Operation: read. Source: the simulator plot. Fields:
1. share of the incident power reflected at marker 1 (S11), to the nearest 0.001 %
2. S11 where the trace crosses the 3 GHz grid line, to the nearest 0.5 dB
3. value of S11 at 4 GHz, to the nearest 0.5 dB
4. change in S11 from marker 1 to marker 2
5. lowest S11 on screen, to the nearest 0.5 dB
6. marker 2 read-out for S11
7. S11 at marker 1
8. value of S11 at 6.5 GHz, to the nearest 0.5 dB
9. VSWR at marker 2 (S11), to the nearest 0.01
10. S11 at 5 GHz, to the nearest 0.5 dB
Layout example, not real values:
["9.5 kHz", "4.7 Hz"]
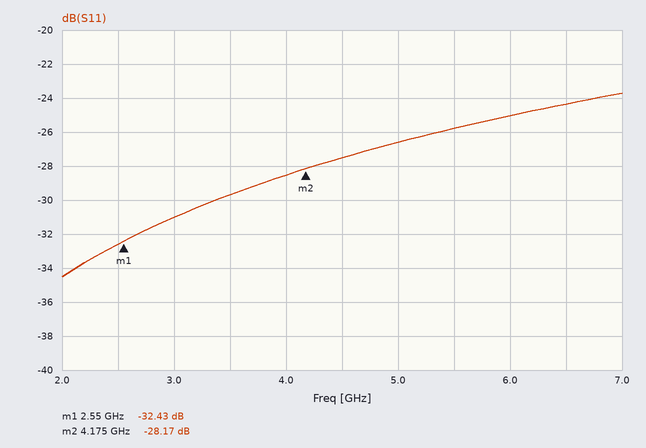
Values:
["0.057 %", "-31.0 dB", "-28.5 dB", "4.26 dB", "-34.5 dB", "-28.17 dB", "-32.43 dB", "-24.5 dB", "1.08", "-26.5 dB"]
